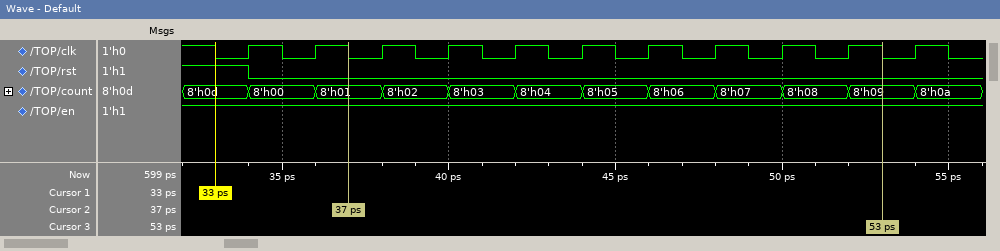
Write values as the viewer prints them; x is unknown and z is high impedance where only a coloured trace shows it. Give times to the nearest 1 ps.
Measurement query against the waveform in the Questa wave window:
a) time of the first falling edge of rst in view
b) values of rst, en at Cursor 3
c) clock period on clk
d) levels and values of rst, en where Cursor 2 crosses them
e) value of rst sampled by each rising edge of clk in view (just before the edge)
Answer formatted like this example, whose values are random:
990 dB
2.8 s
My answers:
34 ps
rst=0, en=1
2 ps
rst=0, en=1
1 0 0 0 0 0 0 0 0 0 0
